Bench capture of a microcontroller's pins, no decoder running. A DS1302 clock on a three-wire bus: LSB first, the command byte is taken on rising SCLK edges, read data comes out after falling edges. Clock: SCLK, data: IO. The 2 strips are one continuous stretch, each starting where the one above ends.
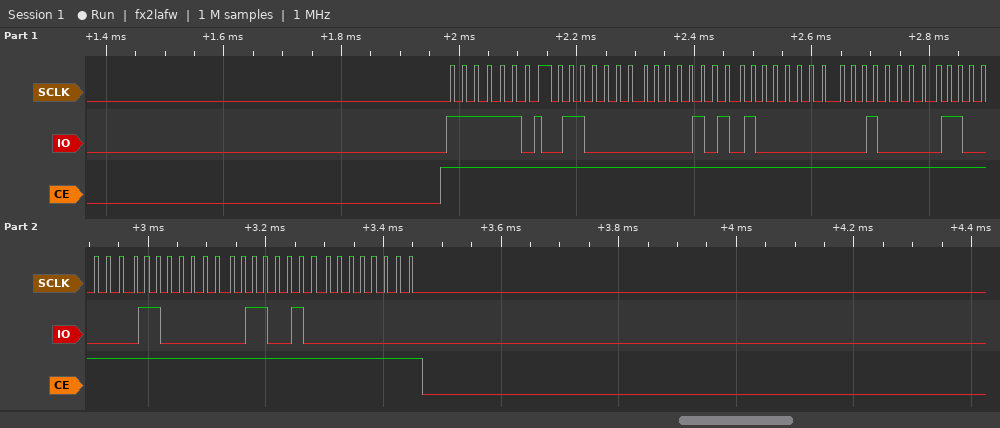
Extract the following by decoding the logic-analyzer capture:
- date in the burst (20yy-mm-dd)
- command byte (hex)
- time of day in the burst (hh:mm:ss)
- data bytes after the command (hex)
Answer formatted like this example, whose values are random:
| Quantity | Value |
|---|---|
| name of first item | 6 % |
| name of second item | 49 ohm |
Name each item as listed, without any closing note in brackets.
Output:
| Quantity | Value |
|---|---|
| date in the burst | 2026-03-04 |
| command byte | 0xBF |
| time of day in the burst | 01:50:06 |
| data bytes after the command | 06 50 01 04 03 03 26 00 |
